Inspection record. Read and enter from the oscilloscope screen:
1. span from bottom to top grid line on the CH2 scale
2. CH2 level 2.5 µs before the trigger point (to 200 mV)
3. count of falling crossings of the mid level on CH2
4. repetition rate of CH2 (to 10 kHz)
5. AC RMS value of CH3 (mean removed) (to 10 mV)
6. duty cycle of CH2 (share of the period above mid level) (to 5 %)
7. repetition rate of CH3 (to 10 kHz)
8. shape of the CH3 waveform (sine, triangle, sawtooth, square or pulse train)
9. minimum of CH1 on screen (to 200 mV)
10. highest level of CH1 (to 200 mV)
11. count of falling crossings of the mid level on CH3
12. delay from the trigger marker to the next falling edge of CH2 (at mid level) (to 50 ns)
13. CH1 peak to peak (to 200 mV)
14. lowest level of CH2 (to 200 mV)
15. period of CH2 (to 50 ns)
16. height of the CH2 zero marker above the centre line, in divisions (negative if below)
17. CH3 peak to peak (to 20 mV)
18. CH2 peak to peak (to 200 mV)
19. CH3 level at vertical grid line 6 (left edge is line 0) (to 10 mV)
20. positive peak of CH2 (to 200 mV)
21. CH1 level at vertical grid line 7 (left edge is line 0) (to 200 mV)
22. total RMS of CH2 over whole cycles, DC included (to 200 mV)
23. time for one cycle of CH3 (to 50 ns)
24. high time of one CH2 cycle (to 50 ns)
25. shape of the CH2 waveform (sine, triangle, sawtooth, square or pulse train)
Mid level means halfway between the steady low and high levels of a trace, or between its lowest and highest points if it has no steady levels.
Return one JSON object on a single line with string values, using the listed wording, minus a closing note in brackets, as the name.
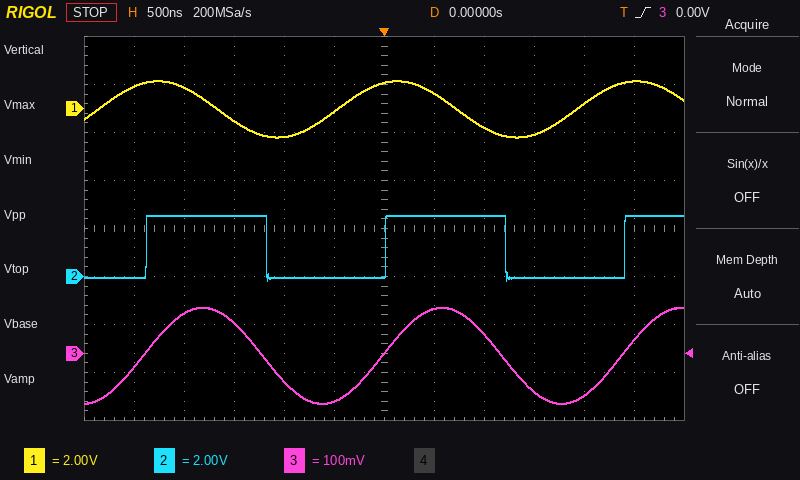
{"span from bottom to top grid line on the CH2 scale": "16 V", "CH2 level 2.5 µs before the trigger point": "0.0 V", "count of falling crossings of the mid level on CH2": "2", "repetition rate of CH2": "420 kHz", "AC RMS value of CH3 (mean removed)": "70 mV", "duty cycle of CH2 (share of the period above mid level)": "50 %", "repetition rate of CH3": "420 kHz", "shape of the CH3 waveform": "sine", "minimum of CH1 on screen": "-1.2 V", "highest level of CH1": "1.2 V", "count of falling crossings of the mid level on CH3": "2", "delay from the trigger marker to the next falling edge of CH2 (at mid level)": "1.20 µs", "CH1 peak to peak": "2.4 V", "lowest level of CH2": "-200 mV", "period of CH2": "2.40 µs", "height of the CH2 zero marker above the centre line, in divisions": "-1.0 div", "CH3 peak to peak": "200 mV", "CH2 peak to peak": "2.8 V", "CH3 level at vertical grid line 6 (left edge is line 0)": "0 mV", "positive peak of CH2": "2.6 V", "CH1 level at vertical grid line 7 (left edge is line 0)": "600 mV", "total RMS of CH2 over whole cycles, DC included": "1.8 V", "time for one cycle of CH3": "2.40 µs", "high time of one CH2 cycle": "1.20 µs", "shape of the CH2 waveform": "square"}
